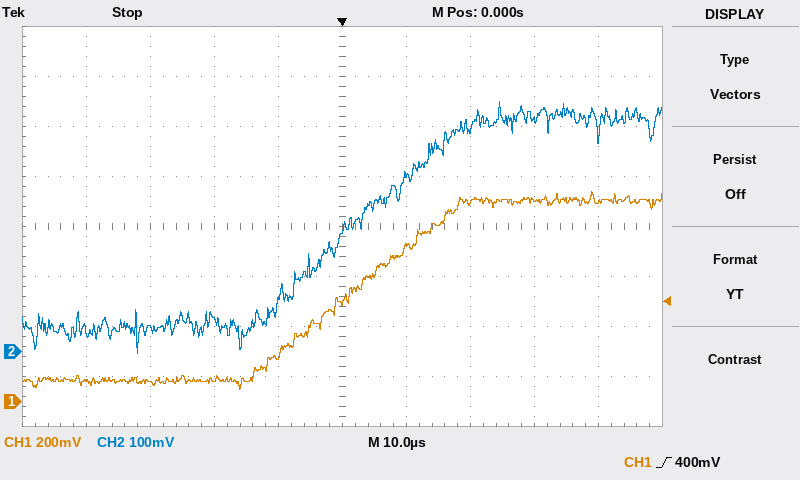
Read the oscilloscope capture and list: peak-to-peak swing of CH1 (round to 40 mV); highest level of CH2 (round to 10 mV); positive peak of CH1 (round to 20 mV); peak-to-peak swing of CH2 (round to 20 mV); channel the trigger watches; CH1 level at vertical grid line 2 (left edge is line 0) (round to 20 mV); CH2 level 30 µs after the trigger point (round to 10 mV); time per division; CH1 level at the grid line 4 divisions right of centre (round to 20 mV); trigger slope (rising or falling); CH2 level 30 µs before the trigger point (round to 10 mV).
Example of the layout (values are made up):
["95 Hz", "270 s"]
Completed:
["800 mV", "500 mV", "840 mV", "500 mV", "CH1", "80 mV", "460 mV", "10 µs", "800 mV", "rising", "40 mV"]
